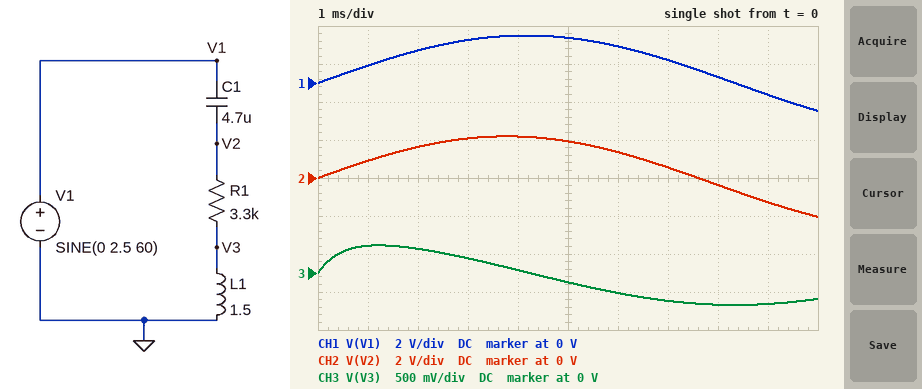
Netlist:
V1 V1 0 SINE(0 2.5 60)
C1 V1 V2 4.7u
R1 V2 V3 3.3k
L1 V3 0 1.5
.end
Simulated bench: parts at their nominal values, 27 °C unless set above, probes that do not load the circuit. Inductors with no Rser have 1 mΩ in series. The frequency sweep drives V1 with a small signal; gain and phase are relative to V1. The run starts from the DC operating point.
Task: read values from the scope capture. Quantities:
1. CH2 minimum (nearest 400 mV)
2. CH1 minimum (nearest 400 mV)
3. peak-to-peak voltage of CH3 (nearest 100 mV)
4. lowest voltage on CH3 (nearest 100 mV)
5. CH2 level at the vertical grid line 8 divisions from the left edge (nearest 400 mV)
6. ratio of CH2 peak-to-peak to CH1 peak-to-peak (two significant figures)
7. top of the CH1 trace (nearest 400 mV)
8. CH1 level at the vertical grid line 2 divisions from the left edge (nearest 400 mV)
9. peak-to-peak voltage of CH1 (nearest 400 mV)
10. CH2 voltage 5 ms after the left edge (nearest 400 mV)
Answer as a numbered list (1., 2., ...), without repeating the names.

1. -2.0 V
2. -1.6 V
3. 800 mV
4. -400 mV
5. -400 mV
6. 1.1
7. 2.4 V
8. 1.6 V
9. 4.0 V
10. 2.0 V
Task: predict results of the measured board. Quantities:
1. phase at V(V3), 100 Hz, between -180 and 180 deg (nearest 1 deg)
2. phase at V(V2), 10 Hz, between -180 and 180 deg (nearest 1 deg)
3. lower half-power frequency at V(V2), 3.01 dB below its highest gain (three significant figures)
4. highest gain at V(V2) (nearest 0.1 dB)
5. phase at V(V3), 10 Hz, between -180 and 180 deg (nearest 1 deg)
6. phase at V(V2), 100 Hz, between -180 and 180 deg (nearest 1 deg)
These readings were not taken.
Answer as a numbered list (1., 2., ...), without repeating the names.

1. 80 deg
2. 47 deg
3. 10.4 Hz
4. 0.2 dB
5. 135 deg
6. 6 deg
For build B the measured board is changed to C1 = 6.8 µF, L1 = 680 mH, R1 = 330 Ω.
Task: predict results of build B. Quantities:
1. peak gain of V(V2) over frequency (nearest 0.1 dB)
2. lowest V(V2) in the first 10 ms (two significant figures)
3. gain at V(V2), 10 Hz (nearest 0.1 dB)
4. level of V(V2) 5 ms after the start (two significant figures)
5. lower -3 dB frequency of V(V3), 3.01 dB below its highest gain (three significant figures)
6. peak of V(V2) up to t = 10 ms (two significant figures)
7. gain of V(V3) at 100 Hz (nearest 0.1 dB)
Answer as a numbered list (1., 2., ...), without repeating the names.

1. 3.2 dB
2. -2.7 V
3. -16.9 dB
4. 760 mV
5. 63.8 Hz
6. 1.7 V
7. 1.0 dB
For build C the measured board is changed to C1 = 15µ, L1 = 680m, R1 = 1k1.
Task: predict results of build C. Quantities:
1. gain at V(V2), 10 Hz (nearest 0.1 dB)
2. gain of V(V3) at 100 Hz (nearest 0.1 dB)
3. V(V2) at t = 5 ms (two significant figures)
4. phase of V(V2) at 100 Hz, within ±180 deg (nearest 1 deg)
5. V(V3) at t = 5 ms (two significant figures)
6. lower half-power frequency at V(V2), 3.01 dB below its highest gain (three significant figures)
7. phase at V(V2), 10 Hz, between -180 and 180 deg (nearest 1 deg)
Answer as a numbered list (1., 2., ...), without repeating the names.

1. -2.7 dB
2. -8.6 dB
3. 2.0 V
4. 5 deg
5. -130 mV
6. 9.83 Hz
7. 45 deg
